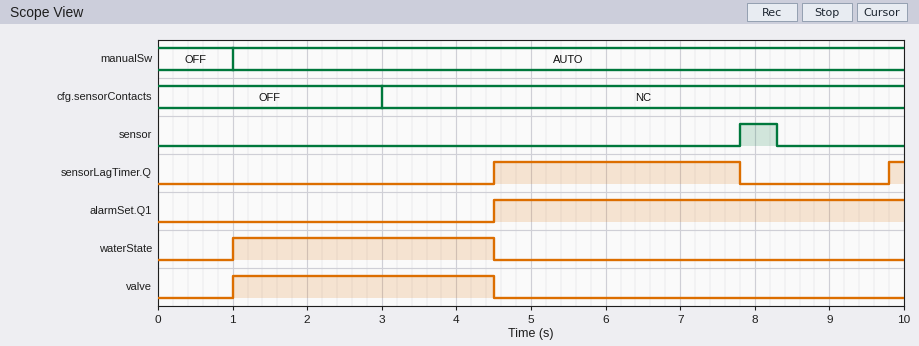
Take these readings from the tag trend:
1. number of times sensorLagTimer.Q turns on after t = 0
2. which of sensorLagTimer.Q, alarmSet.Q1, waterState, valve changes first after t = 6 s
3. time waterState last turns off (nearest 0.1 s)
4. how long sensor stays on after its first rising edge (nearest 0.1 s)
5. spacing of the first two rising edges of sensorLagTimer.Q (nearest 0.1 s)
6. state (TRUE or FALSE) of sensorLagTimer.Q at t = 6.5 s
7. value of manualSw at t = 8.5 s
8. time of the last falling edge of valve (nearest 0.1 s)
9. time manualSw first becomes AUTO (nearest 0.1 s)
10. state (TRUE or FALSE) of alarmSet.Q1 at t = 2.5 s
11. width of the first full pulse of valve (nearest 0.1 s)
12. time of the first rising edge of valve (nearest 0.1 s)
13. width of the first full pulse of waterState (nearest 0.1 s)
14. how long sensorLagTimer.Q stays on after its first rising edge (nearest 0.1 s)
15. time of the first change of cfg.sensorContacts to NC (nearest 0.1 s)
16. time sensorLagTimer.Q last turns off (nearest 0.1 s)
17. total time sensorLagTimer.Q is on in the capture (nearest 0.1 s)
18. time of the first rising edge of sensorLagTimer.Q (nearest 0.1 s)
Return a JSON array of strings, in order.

["2", "sensorLagTimer.Q", "4.5 s", "0.5 s", "5.3 s", "TRUE", "AUTO", "4.5 s", "1.0 s", "FALSE", "3.5 s", "1.0 s", "3.5 s", "3.3 s", "3.0 s", "7.8 s", "3.5 s", "4.5 s"]
